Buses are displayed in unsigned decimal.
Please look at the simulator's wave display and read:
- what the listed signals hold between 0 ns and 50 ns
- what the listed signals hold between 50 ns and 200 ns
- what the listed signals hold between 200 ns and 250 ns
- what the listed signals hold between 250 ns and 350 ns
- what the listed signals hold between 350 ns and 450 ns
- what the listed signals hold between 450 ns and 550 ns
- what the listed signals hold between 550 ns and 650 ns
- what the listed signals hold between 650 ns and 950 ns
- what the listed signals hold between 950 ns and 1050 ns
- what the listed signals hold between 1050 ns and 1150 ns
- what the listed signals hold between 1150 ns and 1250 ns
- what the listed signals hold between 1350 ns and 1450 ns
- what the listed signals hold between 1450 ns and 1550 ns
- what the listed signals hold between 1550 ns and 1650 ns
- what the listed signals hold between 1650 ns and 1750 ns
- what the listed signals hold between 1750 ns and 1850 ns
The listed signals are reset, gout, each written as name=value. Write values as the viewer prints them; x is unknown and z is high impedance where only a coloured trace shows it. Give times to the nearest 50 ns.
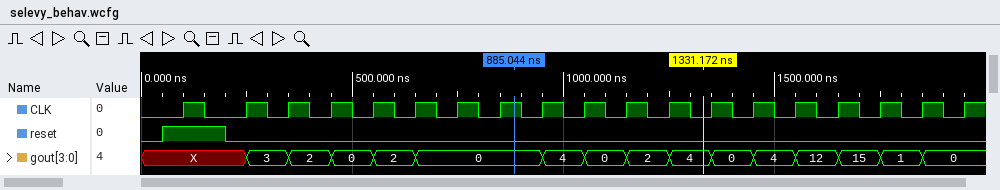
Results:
reset=0, gout=X
reset=1, gout=X
reset=0, gout=X
reset=0, gout=3
reset=0, gout=2
reset=0, gout=0
reset=0, gout=2
reset=0, gout=0
reset=0, gout=4
reset=0, gout=0
reset=0, gout=2
reset=0, gout=0
reset=0, gout=4
reset=0, gout=12
reset=0, gout=15
reset=0, gout=1
